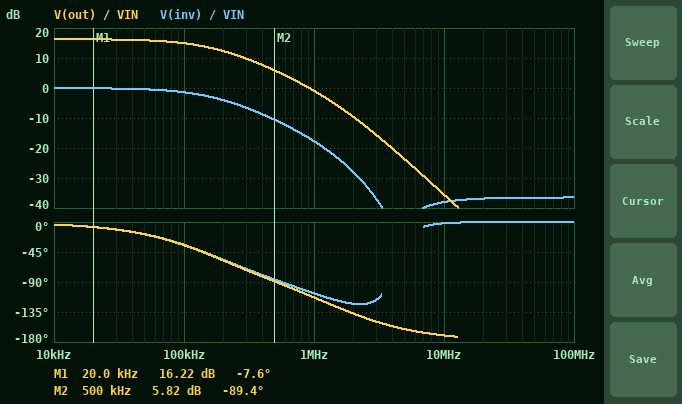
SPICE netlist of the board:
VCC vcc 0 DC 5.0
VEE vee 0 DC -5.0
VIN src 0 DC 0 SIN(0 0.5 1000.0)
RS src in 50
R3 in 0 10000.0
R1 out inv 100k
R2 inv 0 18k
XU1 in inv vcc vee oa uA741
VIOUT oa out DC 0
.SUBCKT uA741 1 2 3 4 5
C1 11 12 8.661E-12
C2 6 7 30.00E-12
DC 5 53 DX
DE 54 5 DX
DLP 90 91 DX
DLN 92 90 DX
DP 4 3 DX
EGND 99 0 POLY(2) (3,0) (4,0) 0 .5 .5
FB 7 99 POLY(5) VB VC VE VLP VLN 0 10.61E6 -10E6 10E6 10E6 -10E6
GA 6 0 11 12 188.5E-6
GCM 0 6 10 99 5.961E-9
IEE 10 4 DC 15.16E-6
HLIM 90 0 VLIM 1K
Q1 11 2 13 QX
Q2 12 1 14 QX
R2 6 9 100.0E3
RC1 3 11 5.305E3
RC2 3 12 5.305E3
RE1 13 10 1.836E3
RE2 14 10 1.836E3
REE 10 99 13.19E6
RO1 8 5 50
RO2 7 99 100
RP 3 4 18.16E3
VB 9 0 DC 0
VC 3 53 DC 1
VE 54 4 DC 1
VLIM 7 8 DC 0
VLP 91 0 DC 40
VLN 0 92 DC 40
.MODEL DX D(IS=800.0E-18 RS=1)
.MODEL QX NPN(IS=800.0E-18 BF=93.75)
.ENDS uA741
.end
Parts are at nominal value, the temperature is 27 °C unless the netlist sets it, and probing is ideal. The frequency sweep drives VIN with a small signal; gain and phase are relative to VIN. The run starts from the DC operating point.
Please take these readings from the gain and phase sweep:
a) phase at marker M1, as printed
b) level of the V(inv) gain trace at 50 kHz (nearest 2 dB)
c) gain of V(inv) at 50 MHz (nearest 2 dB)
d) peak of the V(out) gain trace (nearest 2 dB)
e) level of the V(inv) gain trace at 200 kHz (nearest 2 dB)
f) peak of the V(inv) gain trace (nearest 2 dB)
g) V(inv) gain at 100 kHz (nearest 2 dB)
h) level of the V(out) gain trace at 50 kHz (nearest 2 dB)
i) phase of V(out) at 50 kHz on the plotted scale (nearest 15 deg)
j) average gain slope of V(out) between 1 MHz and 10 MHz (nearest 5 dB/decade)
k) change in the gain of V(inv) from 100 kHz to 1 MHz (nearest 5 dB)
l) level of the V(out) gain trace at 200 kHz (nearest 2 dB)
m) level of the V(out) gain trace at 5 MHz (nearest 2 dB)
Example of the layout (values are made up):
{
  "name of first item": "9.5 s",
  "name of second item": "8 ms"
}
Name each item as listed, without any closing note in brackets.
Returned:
{
  "phase at marker M1, as printed": "-7.6 deg",
  "level of the V(inv) gain trace at 50 kHz": "0 dB",
  "gain of V(inv) at 50 MHz": "-36 dB",
  "peak of the V(out) gain trace": "16 dB",
  "level of the V(inv) gain trace at 200 kHz": "-4 dB",
  "peak of the V(inv) gain trace": "0 dB",
  "V(inv) gain at 100 kHz": "-2 dB",
  "level of the V(out) gain trace at 50 kHz": "16 dB",
  "phase of V(out) at 50 kHz on the plotted scale": "-15 deg",
  "average gain slope of V(out) between 1 MHz and 10 MHz": "-35 dB/decade",
  "change in the gain of V(inv) from 100 kHz to 1 MHz": "-15 dB",
  "level of the V(out) gain trace at 200 kHz": "12 dB",
  "level of the V(out) gain trace at 5 MHz": "-24 dB"
}
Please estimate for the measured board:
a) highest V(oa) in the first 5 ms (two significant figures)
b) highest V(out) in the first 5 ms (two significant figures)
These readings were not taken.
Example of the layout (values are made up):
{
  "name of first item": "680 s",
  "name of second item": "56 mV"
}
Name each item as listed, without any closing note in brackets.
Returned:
{
  "highest V(oa) in the first 5 ms": "3.3 V",
  "highest V(out) in the first 5 ms": "3.3 V"
}
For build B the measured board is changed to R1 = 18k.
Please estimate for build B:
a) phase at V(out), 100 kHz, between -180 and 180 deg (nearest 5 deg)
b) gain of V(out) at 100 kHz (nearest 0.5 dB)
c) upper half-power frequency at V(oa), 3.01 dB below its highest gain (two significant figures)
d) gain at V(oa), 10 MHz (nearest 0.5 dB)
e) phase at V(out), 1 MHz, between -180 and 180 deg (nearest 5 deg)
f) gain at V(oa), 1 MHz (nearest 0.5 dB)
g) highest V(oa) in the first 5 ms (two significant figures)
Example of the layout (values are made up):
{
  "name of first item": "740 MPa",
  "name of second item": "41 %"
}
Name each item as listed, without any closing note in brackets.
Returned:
{
  "phase at V(out), 100 kHz, between -180 and 180 deg": "-10 deg",
  "gain of V(out) at 100 kHz": "6.0 dB",
  "upper half-power frequency at V(oa), 3.01 dB below its highest gain": "650 kHz",
  "gain at V(oa), 10 MHz": "-35.5 dB",
  "phase at V(out), 1 MHz, between -180 and 180 deg": "-95 deg",
  "gain at V(oa), 1 MHz": "0 dB",
  "highest V(oa) in the first 5 ms": "1.0 V"
}
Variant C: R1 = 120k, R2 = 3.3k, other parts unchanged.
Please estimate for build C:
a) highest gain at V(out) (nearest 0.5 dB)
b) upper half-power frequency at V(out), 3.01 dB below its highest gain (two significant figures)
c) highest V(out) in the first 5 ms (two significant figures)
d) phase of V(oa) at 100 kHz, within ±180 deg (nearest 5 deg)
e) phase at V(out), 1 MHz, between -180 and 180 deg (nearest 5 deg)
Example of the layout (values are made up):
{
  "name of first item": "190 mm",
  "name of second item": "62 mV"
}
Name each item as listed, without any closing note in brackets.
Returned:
{
  "highest gain at V(out)": "31.5 dB",
  "upper half-power frequency at V(out), 3.01 dB below its highest gain": "27 kHz",
  "highest V(out) in the first 5 ms": "4.6 V",
  "phase of V(oa) at 100 kHz, within ±180 deg": "-80 deg",
  "phase at V(out), 1 MHz, between -180 and 180 deg": "-120 deg"
}
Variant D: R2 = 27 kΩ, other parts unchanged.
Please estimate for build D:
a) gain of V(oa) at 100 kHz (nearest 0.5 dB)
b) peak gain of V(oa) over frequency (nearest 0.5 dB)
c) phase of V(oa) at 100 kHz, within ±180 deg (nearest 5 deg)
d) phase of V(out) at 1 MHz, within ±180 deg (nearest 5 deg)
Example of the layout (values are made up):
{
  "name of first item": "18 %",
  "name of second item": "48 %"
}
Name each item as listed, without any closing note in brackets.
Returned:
{
  "gain of V(oa) at 100 kHz": "12.5 dB",
  "peak gain of V(oa) over frequency": "13.5 dB",
  "phase of V(oa) at 100 kHz, within ±180 deg": "-25 deg",
  "phase of V(out) at 1 MHz, within ±180 deg": "-110 deg"
}
